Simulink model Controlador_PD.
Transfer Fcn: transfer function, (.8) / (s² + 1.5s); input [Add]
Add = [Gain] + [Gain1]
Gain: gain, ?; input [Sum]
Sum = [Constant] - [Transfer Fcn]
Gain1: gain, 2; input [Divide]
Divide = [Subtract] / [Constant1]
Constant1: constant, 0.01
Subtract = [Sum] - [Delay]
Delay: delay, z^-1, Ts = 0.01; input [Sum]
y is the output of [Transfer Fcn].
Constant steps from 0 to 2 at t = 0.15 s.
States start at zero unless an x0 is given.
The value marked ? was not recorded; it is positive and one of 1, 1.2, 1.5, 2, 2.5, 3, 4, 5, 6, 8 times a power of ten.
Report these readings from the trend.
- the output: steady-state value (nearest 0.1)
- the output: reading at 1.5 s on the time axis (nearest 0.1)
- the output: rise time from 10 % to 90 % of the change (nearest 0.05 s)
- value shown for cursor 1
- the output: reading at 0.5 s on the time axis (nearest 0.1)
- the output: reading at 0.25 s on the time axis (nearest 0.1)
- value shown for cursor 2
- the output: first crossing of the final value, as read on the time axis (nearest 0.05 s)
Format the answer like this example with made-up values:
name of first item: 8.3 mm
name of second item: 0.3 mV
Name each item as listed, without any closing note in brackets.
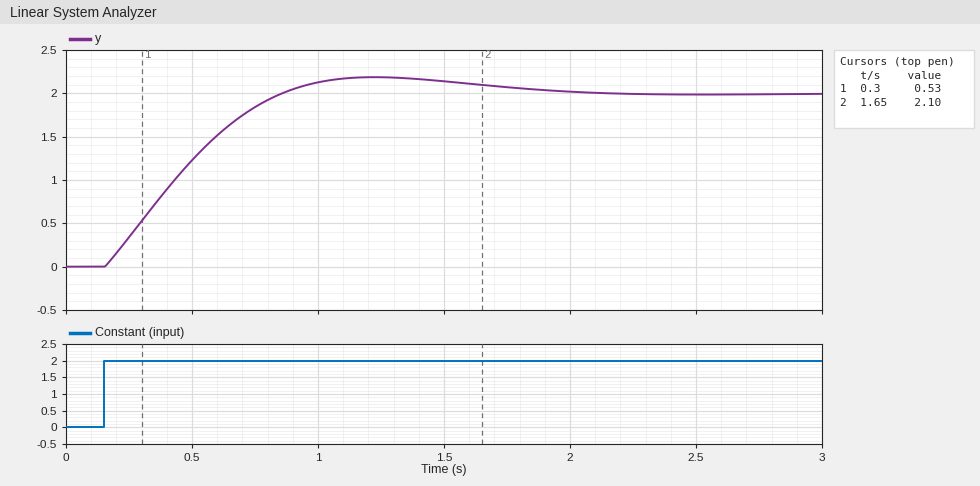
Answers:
the output: steady-state value: 2.0
the output: reading at 1.5 s on the time axis: 2.1
the output: rise time from 10 % to 90 % of the change: 0.50 s
value shown for cursor 1: 0.53
the output: reading at 0.5 s on the time axis: 1.2
the output: reading at 0.25 s on the time axis: 0.3
value shown for cursor 2: 2.10
the output: first crossing of the final value, as read on the time axis: 0.85 s
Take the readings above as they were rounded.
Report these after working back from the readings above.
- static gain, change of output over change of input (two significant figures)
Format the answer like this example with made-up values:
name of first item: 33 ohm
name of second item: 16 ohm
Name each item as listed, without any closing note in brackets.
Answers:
static gain, change of output over change of input: 1.0
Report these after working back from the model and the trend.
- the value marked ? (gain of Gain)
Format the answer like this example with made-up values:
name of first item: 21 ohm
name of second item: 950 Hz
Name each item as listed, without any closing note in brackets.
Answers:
the value marked ?: 12
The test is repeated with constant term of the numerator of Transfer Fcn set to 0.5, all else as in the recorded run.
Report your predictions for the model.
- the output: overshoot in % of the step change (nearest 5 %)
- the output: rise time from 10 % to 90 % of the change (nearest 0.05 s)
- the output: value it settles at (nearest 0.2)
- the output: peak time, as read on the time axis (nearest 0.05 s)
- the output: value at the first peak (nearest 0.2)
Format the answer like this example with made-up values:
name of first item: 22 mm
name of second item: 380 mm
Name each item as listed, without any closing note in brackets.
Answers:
the output: overshoot in % of the step change: 10 %
the output: rise time from 10 % to 90 % of the change: 0.70 s
the output: value it settles at: 2.0
the output: peak time, as read on the time axis: 1.55 s
the output: value at the first peak: 2.2
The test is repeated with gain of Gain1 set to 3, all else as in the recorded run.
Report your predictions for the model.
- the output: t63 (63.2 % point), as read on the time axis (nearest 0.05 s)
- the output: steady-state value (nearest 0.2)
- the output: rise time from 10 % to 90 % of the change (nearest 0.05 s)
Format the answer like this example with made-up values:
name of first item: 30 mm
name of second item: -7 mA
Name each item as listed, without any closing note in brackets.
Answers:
the output: t63 (63.2 % point), as read on the time axis: 0.50 s
the output: steady-state value: 2.0
the output: rise time from 10 % to 90 % of the change: 0.60 s
